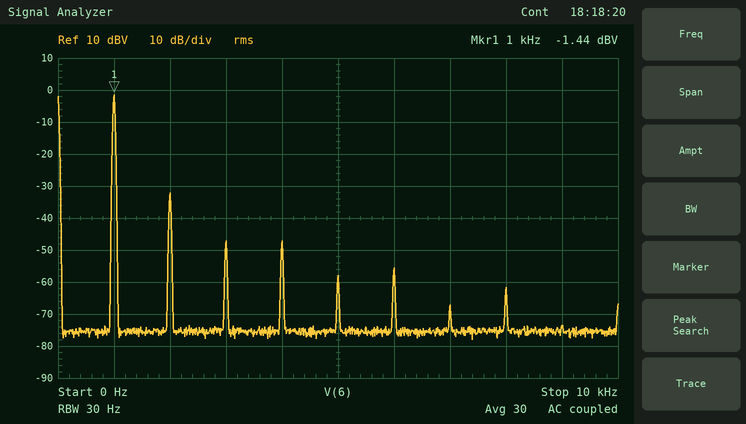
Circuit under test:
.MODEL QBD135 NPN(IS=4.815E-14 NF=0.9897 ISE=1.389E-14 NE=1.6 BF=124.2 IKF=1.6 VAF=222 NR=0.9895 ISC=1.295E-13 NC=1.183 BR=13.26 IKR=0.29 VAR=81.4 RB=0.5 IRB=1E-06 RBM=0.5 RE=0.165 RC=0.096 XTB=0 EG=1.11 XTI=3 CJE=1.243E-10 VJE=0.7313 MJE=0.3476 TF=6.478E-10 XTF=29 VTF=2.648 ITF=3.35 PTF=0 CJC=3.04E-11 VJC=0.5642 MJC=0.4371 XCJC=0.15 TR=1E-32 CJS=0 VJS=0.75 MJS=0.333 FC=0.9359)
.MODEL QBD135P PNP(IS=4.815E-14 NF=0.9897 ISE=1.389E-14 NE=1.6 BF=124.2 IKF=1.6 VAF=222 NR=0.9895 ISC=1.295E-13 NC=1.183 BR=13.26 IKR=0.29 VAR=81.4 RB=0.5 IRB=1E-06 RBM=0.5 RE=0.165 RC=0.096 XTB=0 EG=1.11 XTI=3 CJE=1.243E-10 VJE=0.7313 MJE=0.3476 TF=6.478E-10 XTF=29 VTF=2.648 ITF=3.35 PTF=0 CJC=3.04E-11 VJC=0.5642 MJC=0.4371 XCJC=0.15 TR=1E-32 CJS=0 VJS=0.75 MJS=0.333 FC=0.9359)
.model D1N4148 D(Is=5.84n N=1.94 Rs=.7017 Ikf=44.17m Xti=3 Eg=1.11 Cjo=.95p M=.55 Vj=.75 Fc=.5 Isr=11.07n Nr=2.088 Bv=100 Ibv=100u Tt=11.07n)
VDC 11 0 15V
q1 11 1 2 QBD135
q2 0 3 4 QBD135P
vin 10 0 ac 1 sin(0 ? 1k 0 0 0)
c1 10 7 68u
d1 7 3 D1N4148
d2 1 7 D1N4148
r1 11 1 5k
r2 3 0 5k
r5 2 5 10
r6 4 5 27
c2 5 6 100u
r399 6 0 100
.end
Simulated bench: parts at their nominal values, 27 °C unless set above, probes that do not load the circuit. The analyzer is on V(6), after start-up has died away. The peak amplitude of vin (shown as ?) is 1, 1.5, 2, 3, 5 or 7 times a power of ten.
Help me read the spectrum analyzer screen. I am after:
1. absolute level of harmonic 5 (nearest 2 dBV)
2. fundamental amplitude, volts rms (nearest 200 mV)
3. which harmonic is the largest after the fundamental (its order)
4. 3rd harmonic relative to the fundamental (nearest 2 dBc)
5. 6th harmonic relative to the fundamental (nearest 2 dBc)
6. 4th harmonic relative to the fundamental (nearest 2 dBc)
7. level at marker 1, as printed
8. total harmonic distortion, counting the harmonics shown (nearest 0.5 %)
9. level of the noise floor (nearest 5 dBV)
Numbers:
-58 dBV
800 mV
2
-46 dBc
-54 dBc
-46 dBc
-1.44 dBV
3.0 %
-75 dBV
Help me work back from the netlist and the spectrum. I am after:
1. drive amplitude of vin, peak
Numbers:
1.5 V
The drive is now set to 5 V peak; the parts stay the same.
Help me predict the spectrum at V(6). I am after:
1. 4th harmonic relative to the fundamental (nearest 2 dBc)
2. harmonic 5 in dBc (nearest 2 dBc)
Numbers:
-44 dBc
-48 dBc
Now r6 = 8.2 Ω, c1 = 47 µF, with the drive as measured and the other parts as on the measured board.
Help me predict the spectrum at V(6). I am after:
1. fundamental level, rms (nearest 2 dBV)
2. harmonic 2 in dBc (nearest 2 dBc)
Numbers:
0 dBV
-50 dBc
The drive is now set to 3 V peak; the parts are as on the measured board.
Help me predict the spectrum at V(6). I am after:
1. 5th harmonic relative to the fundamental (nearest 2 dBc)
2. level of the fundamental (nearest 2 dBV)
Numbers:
-52 dBc
4 dBV
